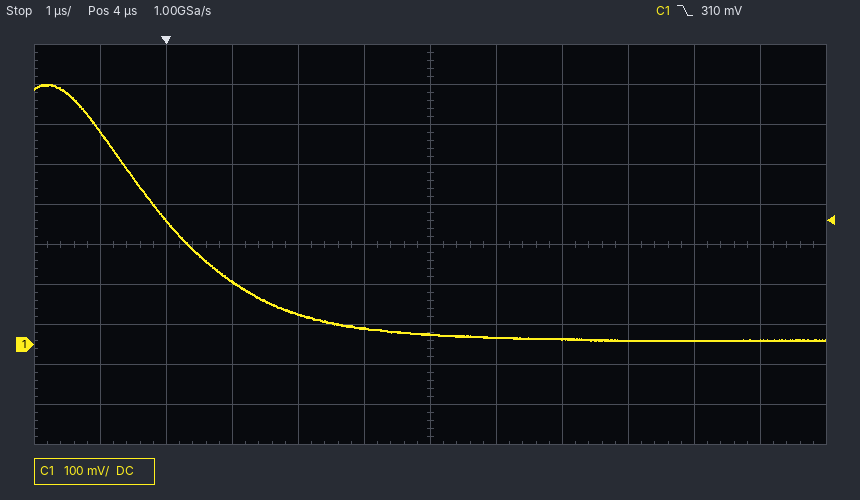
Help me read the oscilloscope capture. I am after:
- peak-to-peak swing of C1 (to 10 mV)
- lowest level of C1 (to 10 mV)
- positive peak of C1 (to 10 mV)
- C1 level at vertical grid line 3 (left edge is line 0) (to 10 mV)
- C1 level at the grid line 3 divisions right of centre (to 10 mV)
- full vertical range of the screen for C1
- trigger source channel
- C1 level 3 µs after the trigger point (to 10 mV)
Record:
640 mV
10 mV
650 mV
160 mV
10 mV
1 V
C1
40 mV
